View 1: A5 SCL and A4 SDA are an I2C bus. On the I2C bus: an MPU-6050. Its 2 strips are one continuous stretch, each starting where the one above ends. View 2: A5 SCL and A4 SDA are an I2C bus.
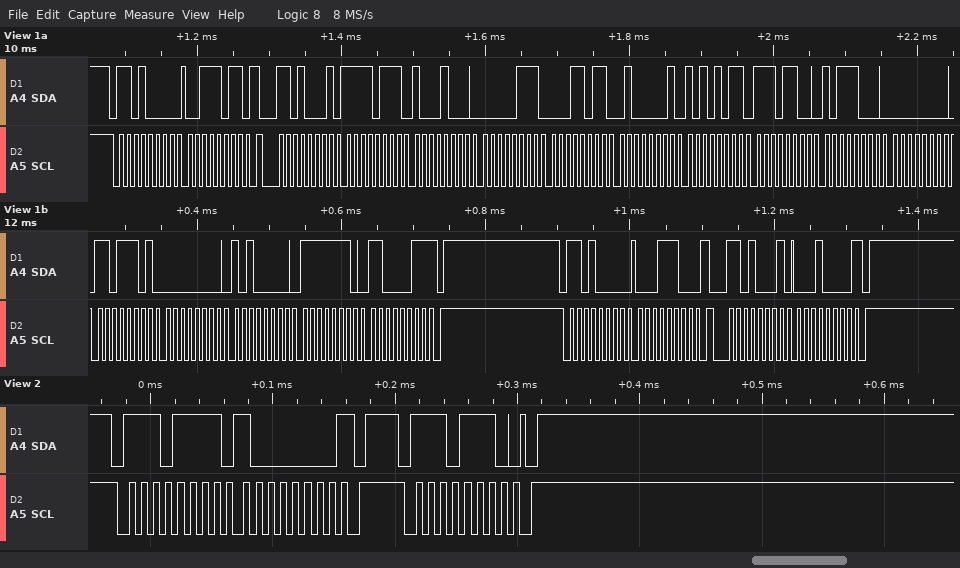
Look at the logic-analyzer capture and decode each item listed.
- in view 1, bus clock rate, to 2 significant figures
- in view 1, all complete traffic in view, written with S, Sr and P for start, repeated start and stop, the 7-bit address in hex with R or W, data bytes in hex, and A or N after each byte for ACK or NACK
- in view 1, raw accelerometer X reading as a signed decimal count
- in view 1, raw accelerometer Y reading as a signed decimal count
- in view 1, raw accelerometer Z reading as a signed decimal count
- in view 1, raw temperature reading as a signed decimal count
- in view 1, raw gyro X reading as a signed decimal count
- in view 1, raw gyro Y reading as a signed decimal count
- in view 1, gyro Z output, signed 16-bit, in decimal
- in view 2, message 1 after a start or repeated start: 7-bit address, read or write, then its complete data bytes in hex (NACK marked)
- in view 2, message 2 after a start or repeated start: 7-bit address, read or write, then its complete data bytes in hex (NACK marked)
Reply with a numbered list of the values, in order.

1. 100 kHz
2. S 68W A 3B A Sr 68R A F7 A 88 A 07 A 1B A 41 A AB A EC A B8 A 00 A DD A 00 A A0 A FE A C3 N P S 68W A 1C A Sr 68R A 10 N P
3. -2168
4. 1819
5. 16811
6. -4936
7. 221
8. 160
9. -317
10. 0x77 read: 80 NACK
11. 0x77 write
